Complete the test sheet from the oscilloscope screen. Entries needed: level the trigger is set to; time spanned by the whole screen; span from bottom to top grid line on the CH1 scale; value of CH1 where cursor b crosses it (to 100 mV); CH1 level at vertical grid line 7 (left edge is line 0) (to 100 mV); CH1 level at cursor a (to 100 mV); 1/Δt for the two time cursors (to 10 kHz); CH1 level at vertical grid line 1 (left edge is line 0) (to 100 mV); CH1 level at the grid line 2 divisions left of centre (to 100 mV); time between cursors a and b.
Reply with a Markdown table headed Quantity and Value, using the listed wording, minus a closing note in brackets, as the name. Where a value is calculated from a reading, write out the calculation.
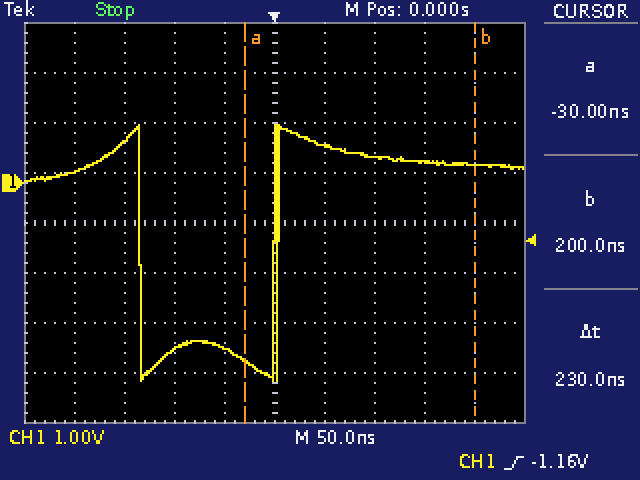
| Quantity | Value |
|---|---|
| level the trigger is set to | -1.16 V |
| time spanned by the whole screen | 500 ns |
| span from bottom to top grid line on the CH1 scale | 8 V |
| value of CH1 where cursor b crosses it | 400 mV |
| CH1 level at vertical grid line 7 (left edge is line 0) | 500 mV |
| CH1 level at cursor a | -3.6 V |
| 1/Δt for the two time cursors | 1 / 230 ns ≈ 4.35 MHz |
| CH1 level at vertical grid line 1 (left edge is line 0) | 200 mV |
| CH1 level at the grid line 2 divisions left of centre | -3.3 V |
| time between cursors a and b | 230 ns |
